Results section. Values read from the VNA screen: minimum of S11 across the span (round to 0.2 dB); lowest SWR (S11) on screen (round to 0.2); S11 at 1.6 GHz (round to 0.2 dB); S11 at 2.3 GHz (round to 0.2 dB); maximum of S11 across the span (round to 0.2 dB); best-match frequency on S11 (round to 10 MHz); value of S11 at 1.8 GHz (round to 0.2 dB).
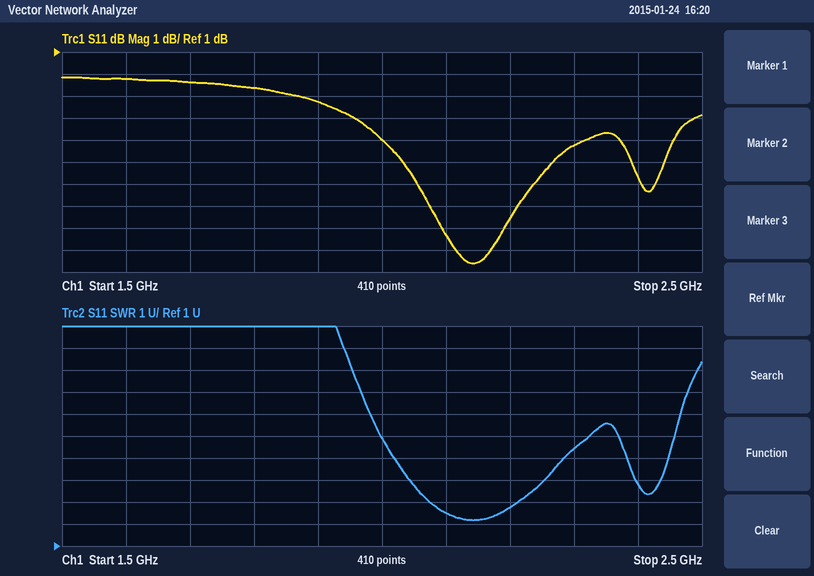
-8.6 dB
2.2
-0.2 dB
-3.2 dB
-0.2 dB
2.14 GHz
-0.6 dB
